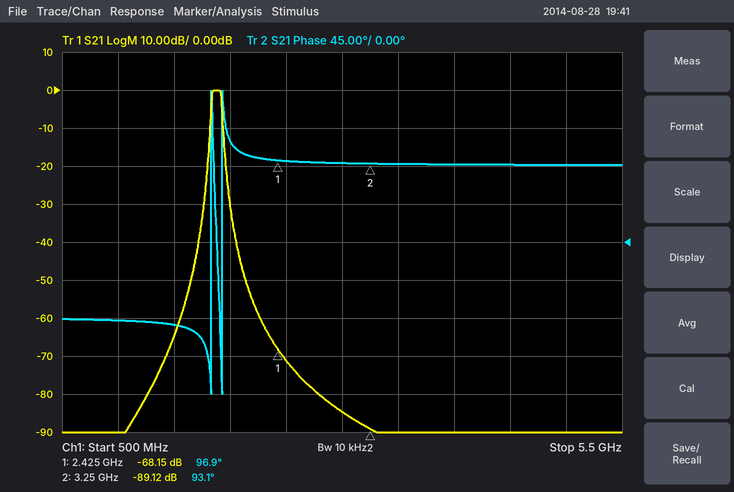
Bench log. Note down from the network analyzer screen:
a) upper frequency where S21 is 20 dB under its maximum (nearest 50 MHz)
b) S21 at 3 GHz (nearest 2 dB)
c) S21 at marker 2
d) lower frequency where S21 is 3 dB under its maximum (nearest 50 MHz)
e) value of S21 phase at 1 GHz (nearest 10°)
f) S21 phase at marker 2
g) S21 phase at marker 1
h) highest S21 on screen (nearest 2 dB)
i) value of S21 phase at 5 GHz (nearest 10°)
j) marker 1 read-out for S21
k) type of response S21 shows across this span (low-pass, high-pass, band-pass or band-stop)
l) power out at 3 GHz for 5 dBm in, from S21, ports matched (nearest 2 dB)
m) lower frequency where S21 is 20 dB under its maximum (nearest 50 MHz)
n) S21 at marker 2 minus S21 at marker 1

1.95 GHz
-84 dB
-89.12 dB
1.85 GHz
-90°
93.1°
96.9°
0 dB
90°
-68.15 dB
band-pass
-80 dBm
1.80 GHz
-20.97 dB
